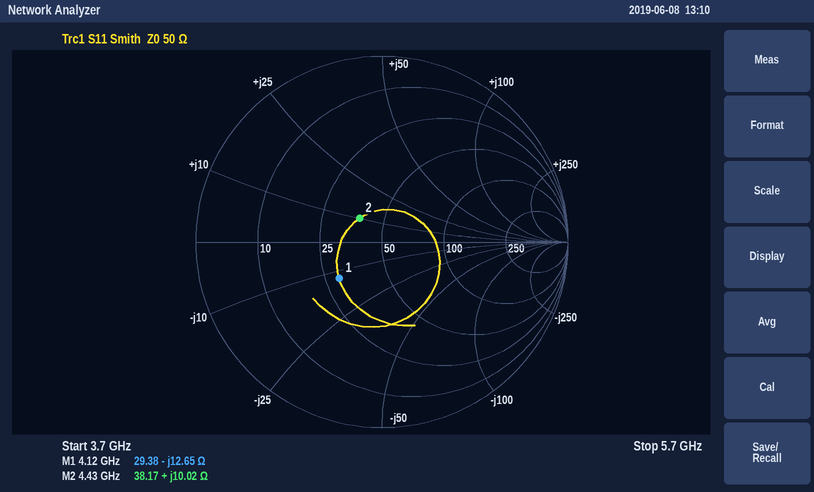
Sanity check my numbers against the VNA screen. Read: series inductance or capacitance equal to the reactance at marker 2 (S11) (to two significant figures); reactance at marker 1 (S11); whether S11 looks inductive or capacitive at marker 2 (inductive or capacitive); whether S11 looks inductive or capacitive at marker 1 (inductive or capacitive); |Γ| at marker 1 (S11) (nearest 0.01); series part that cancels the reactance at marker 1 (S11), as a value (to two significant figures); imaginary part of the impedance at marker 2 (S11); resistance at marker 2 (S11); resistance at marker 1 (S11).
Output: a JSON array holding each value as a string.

["360 pH", "-12.65 Ω", "inductive", "capacitive", "0.30", "490 pH", "+10.02 Ω", "38.17 Ω", "29.38 Ω"]
